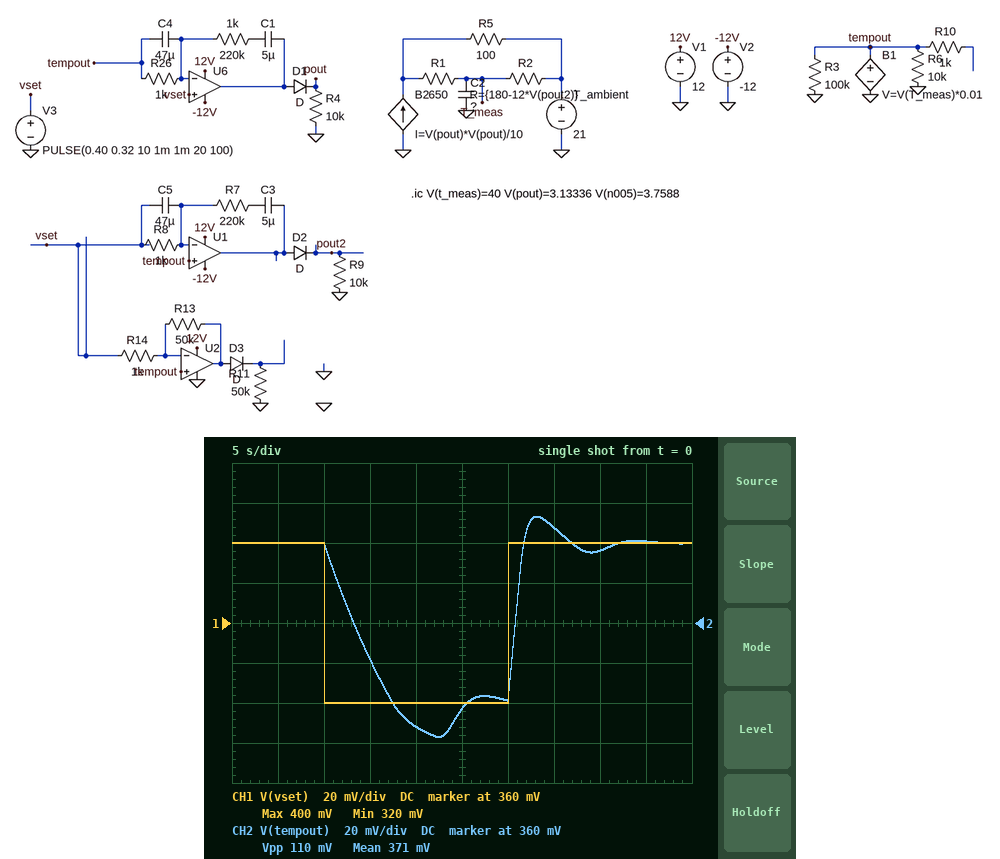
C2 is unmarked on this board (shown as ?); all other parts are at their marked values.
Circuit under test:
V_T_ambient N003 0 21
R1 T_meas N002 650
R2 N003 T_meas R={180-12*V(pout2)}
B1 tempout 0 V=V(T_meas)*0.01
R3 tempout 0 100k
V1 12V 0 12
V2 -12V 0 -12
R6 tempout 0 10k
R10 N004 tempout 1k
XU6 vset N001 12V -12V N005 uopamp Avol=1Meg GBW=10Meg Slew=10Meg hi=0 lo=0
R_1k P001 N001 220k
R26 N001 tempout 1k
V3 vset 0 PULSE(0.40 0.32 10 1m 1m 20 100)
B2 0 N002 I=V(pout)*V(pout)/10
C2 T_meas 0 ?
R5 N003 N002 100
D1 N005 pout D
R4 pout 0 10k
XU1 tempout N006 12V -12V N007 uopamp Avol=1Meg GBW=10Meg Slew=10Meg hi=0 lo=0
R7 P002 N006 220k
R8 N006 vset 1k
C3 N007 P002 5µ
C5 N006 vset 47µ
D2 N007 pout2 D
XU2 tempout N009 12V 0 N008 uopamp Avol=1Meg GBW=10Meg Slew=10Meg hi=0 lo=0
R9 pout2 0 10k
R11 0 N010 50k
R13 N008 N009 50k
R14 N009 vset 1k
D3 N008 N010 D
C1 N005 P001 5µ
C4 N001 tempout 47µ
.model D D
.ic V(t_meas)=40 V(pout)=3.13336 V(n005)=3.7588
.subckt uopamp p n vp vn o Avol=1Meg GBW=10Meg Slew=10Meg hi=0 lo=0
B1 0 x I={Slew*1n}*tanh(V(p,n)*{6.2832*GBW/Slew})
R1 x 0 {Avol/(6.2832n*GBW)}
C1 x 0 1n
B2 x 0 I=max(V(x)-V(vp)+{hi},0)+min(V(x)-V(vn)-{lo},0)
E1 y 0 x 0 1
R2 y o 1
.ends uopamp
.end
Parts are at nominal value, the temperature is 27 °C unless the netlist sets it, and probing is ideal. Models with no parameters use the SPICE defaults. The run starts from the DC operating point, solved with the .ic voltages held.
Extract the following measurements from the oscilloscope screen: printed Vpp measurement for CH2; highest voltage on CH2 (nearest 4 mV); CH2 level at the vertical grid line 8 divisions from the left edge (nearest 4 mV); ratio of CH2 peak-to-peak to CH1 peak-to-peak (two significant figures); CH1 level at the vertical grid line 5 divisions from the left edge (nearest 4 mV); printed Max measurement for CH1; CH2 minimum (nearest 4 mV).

110 mV
412 mV
396 mV
1.4
320 mV
400 mV
304 mV
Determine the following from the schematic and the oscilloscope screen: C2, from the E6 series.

330 mF
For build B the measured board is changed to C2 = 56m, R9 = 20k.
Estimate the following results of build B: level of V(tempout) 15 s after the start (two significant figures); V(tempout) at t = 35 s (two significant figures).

320 mV
400 mV
